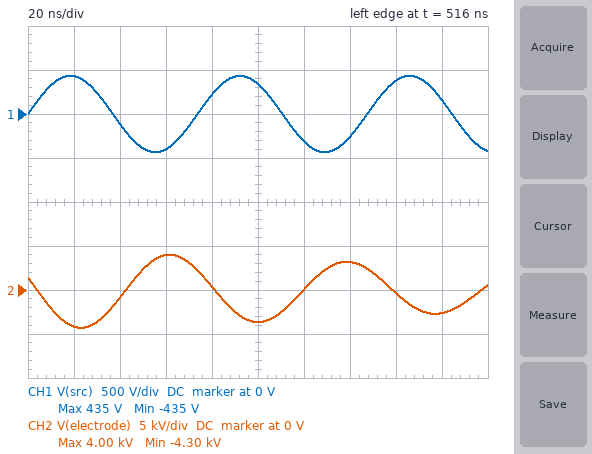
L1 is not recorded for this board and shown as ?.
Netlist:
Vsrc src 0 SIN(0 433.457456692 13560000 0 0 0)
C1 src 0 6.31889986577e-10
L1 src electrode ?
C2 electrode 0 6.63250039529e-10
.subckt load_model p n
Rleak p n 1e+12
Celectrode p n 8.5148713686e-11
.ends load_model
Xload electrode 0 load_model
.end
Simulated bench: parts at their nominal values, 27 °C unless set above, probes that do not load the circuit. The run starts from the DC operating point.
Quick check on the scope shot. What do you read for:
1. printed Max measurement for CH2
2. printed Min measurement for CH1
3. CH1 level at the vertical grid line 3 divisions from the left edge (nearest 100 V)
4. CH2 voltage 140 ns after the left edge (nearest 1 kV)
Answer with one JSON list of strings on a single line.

["4.00 kV", "-435 V", "-400 V", "3 kV"]
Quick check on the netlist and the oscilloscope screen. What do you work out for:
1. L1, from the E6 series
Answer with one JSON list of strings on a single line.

["220 nH"]
